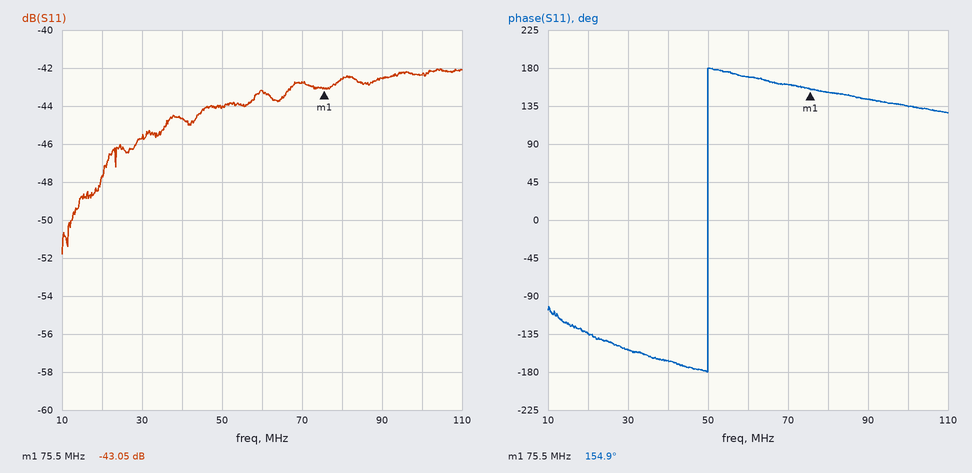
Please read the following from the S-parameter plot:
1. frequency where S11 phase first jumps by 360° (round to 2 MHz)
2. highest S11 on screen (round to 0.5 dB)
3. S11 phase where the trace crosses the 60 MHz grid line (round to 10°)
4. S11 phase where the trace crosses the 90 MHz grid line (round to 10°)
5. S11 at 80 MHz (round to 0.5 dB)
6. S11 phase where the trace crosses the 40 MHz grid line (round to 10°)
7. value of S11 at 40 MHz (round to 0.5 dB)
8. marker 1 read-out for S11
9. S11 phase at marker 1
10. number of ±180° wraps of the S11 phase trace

50 MHz
-42.0 dB
170°
140°
-42.5 dB
-170°
-44.5 dB
-43.05 dB
154.9°
1
